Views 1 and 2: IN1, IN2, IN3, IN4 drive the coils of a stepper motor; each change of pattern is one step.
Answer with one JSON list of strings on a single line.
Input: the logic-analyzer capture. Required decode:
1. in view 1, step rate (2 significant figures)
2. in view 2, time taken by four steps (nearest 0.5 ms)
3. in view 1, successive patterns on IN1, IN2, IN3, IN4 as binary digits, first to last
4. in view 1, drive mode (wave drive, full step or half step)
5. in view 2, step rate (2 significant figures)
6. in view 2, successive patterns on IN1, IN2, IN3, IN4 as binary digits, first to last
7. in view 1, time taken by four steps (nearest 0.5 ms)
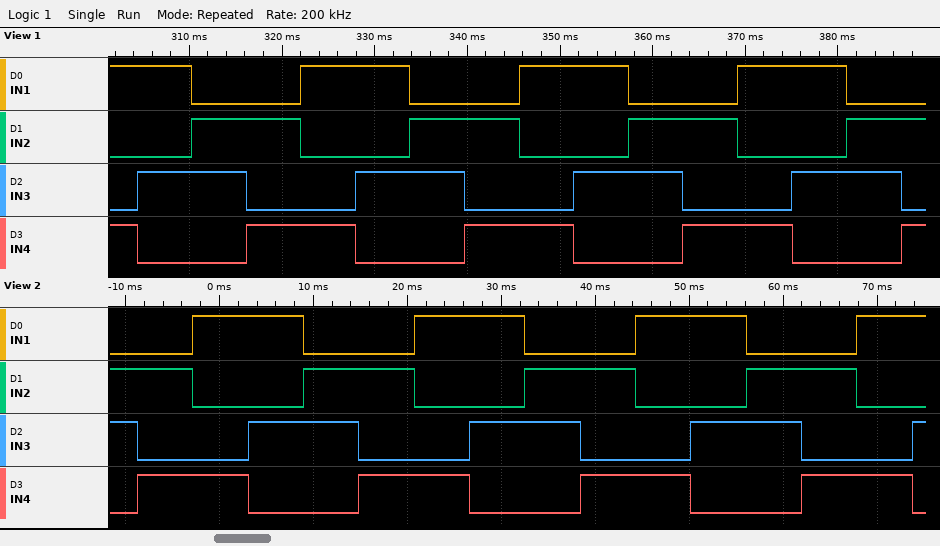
["170 steps/s", "23.5 ms", "1001 1010 0110 0101 1001 1010 0110 0101 1001 1010 0110 0101 1001 1010 0110 0101", "full step", "170 steps/s", "0110 0101 1001 1010 0110 0101 1001 1010 0110 0101 1001 1010 0110 0101 1001 1010", "23.5 ms"]
